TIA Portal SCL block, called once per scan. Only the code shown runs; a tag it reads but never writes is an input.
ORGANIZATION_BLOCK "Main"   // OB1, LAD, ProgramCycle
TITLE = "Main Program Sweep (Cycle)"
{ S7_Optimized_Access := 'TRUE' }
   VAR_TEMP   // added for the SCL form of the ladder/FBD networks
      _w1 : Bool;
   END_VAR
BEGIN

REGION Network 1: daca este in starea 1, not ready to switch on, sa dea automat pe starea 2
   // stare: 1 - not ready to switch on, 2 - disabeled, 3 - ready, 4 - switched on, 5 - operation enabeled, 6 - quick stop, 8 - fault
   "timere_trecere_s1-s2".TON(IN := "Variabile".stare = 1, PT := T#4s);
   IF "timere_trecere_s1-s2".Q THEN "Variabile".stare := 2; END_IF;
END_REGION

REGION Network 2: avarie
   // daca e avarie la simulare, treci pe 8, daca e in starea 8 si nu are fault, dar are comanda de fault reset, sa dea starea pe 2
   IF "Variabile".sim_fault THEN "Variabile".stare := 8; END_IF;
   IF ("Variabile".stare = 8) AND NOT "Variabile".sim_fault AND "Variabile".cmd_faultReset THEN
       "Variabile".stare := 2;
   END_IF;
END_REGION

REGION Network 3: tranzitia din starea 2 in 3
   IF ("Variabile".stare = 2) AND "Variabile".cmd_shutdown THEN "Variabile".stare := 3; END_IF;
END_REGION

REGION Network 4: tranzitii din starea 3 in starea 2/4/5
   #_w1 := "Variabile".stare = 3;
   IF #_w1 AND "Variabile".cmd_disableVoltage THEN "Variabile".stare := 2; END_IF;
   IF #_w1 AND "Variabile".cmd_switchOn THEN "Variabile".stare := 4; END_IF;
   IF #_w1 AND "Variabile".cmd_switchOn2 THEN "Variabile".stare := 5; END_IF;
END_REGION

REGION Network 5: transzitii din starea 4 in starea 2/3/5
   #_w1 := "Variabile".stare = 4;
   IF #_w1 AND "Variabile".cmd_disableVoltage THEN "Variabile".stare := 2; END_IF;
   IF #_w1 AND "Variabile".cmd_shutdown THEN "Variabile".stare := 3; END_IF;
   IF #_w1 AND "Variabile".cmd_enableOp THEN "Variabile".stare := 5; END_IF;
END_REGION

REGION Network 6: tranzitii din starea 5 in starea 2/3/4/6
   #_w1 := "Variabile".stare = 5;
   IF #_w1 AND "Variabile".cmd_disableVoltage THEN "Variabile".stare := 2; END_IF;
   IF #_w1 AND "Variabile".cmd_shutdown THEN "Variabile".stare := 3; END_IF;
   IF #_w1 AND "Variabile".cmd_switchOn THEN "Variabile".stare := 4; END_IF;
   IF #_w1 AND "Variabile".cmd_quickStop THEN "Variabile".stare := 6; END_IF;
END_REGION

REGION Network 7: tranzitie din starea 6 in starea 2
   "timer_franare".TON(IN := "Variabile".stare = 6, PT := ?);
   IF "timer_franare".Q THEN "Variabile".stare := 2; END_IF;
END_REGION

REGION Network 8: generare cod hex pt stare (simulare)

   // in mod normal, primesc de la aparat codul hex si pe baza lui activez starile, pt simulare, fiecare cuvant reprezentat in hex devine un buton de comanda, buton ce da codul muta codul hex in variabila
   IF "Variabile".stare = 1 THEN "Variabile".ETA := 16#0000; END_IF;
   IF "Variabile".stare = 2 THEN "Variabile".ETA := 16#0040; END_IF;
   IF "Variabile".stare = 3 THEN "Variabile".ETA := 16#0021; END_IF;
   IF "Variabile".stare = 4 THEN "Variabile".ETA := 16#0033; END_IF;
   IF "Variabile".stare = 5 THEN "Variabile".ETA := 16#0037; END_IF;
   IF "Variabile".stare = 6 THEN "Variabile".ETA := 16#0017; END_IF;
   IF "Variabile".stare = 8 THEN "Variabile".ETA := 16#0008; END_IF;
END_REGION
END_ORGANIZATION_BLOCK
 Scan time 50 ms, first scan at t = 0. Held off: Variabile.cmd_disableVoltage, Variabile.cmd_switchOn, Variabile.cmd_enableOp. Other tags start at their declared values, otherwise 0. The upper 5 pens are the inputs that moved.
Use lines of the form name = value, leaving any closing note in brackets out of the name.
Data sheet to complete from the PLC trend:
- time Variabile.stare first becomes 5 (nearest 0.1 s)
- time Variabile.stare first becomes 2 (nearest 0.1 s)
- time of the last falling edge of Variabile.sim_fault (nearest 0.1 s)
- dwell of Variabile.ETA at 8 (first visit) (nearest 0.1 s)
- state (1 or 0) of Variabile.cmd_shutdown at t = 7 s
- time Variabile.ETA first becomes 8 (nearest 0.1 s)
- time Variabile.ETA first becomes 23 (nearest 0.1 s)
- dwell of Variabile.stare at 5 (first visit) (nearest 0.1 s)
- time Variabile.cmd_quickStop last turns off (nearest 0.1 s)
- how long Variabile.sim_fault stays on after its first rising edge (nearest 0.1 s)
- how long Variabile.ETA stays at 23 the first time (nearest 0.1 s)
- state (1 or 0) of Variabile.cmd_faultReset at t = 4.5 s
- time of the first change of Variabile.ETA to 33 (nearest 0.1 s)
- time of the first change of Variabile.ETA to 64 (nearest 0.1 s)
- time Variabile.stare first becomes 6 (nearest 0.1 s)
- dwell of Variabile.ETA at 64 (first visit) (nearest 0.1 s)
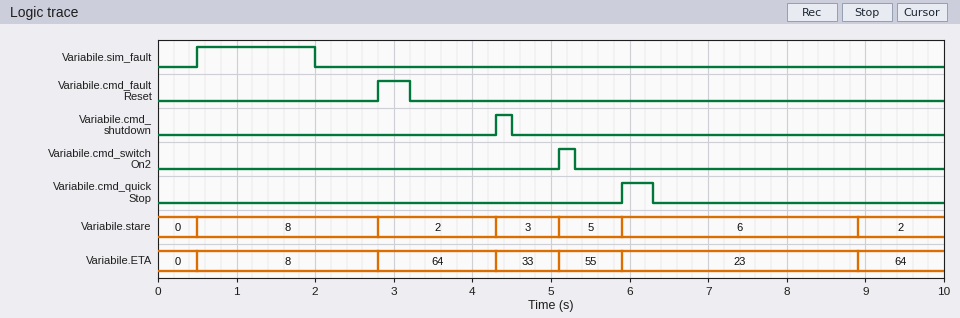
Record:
time Variabile.stare first becomes 5 = 5.1 s
time Variabile.stare first becomes 2 = 2.8 s
time of the last falling edge of Variabile.sim_fault = 2.0 s
dwell of Variabile.ETA at 8 (first visit) = 2.3 s
state (1 or 0) of Variabile.cmd_shutdown at t = 7 s = 0
time Variabile.ETA first becomes 8 = 0.5 s
time Variabile.ETA first becomes 23 = 5.9 s
dwell of Variabile.stare at 5 (first visit) = 0.8 s
time Variabile.cmd_quickStop last turns off = 6.3 s
how long Variabile.sim_fault stays on after its first rising edge = 1.5 s
how long Variabile.ETA stays at 23 the first time = 3.0 s
state (1 or 0) of Variabile.cmd_faultReset at t = 4.5 s = 0
time of the first change of Variabile.ETA to 33 = 4.3 s
time of the first change of Variabile.ETA to 64 = 2.8 s
time Variabile.stare first becomes 6 = 5.9 s
dwell of Variabile.ETA at 64 (first visit) = 1.5 s
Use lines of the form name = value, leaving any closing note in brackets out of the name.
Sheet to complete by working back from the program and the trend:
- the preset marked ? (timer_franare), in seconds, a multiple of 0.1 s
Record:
the preset marked ? (timer_franare), in seconds, a multiple of 0.1 s = 3.0 s
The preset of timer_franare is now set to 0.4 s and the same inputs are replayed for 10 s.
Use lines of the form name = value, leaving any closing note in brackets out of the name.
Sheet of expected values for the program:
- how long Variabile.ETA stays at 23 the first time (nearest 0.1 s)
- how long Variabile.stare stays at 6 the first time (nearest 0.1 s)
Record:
how long Variabile.ETA stays at 23 the first time = 0.4 s
how long Variabile.stare stays at 6 the first time = 0.4 s
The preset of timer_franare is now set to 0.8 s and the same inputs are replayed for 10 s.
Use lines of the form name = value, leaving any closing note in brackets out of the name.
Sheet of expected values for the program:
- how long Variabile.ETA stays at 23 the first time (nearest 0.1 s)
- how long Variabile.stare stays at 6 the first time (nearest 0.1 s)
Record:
how long Variabile.ETA stays at 23 the first time = 0.8 s
how long Variabile.stare stays at 6 the first time = 0.8 s
